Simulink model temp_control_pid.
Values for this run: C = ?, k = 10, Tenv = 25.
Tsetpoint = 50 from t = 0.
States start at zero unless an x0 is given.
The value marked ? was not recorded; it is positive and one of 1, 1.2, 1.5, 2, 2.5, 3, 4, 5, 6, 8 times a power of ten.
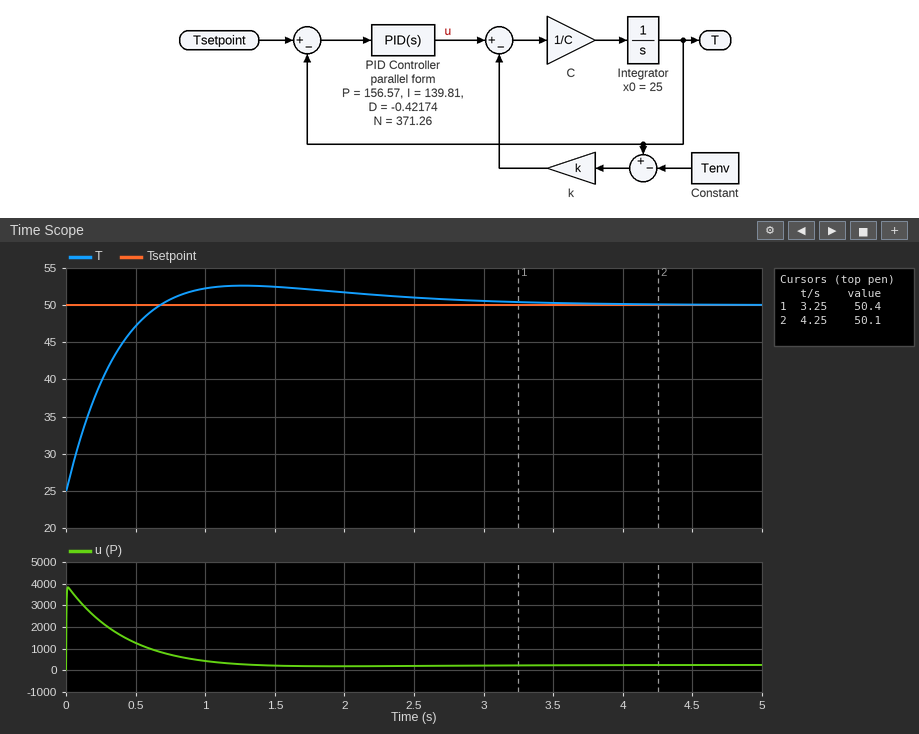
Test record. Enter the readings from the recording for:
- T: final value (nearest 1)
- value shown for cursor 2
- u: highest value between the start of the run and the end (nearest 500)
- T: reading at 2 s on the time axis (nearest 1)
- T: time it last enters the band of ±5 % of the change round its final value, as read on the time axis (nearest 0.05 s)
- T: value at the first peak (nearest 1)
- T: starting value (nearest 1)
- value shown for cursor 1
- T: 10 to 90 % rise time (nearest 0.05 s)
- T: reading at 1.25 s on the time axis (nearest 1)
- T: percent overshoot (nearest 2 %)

50
50.1
4000
52
2.30 s
53
25
50.4
0.50 s
53
10 %
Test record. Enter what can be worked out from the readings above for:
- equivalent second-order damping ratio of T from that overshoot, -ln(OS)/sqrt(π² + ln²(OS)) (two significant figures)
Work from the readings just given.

0.59
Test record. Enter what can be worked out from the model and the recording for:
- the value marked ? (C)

50
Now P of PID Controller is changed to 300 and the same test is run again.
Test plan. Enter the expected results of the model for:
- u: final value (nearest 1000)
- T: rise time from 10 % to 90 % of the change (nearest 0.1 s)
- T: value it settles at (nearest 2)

0
0.3 s
50
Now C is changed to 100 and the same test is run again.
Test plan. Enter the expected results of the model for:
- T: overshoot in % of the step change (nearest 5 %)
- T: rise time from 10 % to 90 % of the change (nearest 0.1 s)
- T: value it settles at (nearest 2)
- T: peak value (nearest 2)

20 %
0.8 s
50
54
